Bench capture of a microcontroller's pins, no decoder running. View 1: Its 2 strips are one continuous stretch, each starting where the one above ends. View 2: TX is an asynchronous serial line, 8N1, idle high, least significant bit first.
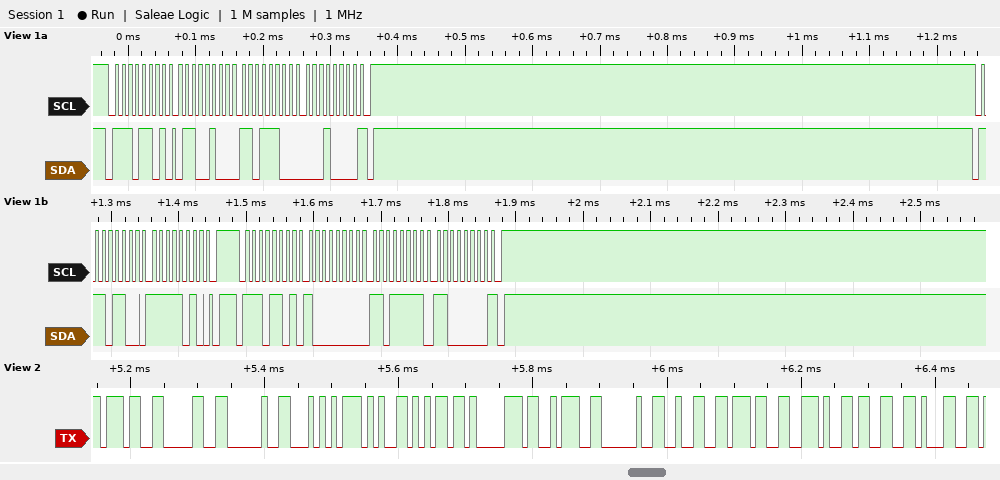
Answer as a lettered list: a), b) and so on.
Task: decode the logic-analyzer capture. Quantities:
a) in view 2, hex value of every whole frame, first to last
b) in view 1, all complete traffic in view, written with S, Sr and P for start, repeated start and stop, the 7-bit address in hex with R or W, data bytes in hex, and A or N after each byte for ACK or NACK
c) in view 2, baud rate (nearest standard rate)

a) 37 30 20 54 65 6D 70 3A 20 32 37 2E 33 31
b) S 76R A 64 A DC A 10 N P S 76W A FA A P S 76R A 80 A DF A C0 N P
c) 115200 baud
